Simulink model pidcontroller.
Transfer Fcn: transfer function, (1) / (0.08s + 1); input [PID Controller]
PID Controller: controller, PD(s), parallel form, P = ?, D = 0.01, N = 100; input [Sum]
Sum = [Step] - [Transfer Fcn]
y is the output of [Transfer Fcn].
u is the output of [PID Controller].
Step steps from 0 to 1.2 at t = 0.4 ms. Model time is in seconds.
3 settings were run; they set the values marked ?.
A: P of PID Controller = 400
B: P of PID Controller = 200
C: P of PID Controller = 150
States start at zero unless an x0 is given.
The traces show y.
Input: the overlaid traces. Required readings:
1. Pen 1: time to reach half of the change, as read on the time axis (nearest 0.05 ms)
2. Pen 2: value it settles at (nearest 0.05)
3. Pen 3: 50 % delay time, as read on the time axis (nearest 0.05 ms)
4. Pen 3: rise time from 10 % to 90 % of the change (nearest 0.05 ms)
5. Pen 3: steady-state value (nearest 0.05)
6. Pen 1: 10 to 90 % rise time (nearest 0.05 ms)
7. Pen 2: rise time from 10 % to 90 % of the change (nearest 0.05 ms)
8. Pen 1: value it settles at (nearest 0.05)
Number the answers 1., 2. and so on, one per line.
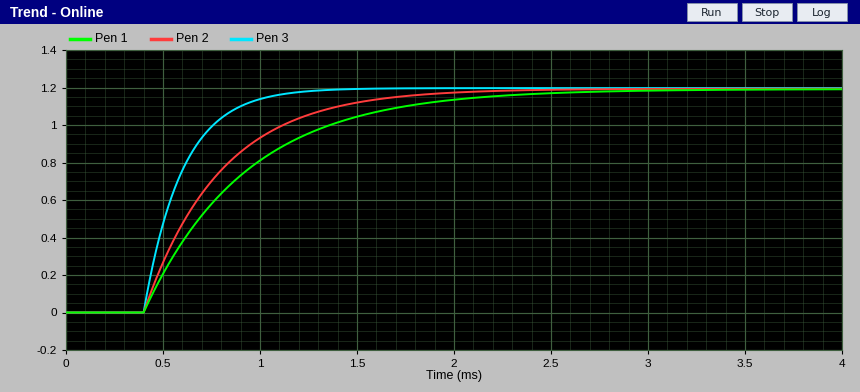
1. 0.75 ms
2. 1.20
3. 0.55 ms
4. 0.45 ms
5. 1.20
6. 1.15 ms
7. 0.85 ms
8. 1.20
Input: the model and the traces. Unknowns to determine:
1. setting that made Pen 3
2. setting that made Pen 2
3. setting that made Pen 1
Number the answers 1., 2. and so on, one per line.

1. A
2. B
3. C
